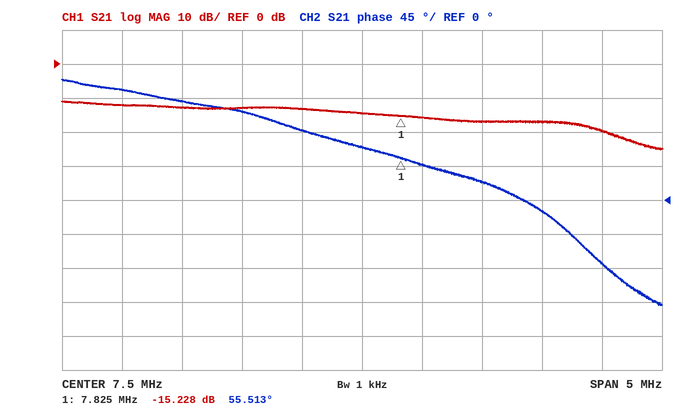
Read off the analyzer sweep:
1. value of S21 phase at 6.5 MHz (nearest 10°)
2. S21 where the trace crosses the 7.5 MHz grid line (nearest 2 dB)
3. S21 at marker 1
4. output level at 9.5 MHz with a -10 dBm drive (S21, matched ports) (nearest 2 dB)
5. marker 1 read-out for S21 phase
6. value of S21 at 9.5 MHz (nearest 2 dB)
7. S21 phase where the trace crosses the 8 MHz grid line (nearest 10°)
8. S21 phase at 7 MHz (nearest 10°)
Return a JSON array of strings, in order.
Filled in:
["120°", "-14 dB", "-15.228 dB", "-30 dBm", "55.513°", "-20 dB", "50°", "90°"]
